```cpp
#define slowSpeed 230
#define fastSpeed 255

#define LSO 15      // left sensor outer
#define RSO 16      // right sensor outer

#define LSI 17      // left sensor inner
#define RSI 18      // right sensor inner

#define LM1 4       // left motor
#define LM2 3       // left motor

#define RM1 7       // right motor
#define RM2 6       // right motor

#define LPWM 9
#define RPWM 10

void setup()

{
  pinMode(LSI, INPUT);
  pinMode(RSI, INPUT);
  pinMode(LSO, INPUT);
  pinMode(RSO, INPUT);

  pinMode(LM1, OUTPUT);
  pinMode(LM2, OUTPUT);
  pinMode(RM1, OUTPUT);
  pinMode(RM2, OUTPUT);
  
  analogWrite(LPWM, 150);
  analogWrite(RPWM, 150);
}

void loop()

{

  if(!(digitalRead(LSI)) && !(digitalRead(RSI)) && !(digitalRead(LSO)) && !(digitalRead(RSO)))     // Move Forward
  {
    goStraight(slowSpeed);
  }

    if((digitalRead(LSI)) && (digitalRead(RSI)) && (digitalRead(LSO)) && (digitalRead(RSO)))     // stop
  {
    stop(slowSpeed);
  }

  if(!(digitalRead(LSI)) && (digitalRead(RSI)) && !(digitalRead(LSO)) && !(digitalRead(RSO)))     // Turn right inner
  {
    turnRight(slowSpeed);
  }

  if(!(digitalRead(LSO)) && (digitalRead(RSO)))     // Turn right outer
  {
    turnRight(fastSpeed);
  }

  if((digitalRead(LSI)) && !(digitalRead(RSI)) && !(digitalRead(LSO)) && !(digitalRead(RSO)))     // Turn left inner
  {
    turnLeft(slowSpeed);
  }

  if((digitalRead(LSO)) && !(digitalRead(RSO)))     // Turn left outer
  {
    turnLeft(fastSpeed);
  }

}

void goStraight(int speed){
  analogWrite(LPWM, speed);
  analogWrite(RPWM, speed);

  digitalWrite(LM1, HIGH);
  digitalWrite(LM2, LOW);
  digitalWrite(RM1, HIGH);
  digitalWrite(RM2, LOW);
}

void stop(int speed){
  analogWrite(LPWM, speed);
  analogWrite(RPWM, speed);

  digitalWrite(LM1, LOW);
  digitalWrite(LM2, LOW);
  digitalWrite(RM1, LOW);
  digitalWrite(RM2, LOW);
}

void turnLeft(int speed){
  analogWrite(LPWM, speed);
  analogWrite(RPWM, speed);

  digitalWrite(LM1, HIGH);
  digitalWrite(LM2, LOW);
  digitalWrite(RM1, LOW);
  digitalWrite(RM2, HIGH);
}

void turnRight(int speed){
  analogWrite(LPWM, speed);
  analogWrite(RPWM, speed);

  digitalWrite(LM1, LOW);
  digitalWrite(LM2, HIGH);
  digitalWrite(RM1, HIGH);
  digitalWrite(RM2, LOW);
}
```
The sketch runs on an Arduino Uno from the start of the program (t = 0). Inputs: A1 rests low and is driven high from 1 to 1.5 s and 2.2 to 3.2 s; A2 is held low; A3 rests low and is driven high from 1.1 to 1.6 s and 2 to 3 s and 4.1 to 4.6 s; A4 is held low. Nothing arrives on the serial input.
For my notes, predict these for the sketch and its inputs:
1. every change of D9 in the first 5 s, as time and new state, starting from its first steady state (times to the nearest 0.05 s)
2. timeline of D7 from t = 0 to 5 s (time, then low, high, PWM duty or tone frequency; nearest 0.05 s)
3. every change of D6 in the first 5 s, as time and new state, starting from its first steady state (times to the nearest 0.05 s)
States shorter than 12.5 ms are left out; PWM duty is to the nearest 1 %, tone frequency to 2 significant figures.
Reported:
0 s PWM 90 %; 1 s high; 1.5 s PWM 90 %; 2.2 s high; 3.2 s PWM 90 %
0 s high; 1 s low; 1.6 s high; 2 s low; 3.2 s high; 4.1 s low; 4.6 s high
0 s low; 1 s high; 1.6 s low; 2 s high; 3.2 s low; 4.1 s high; 4.6 s low
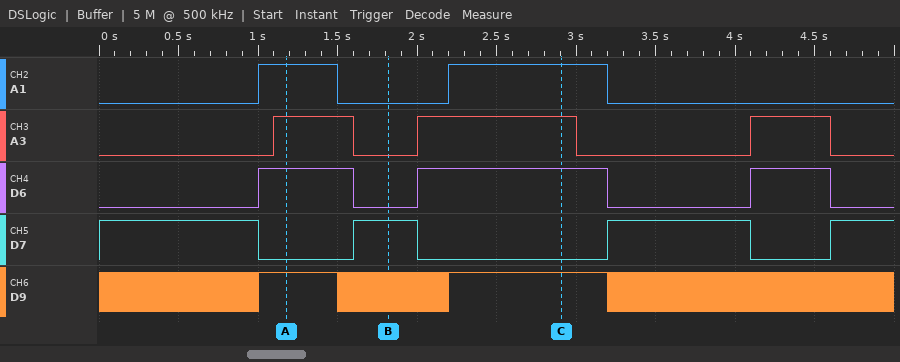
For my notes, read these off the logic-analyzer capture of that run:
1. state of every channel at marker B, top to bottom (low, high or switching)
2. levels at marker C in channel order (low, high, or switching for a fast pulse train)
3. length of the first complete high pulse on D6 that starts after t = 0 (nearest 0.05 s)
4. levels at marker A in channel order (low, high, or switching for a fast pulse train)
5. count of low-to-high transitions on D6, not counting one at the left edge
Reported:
A1 low, A3 low, D6 low, D7 high, D9 switching
A1 high, A3 high, D6 high, D7 low, D9 high
0.60 s
A1 high, A3 high, D6 high, D7 low, D9 high
3
